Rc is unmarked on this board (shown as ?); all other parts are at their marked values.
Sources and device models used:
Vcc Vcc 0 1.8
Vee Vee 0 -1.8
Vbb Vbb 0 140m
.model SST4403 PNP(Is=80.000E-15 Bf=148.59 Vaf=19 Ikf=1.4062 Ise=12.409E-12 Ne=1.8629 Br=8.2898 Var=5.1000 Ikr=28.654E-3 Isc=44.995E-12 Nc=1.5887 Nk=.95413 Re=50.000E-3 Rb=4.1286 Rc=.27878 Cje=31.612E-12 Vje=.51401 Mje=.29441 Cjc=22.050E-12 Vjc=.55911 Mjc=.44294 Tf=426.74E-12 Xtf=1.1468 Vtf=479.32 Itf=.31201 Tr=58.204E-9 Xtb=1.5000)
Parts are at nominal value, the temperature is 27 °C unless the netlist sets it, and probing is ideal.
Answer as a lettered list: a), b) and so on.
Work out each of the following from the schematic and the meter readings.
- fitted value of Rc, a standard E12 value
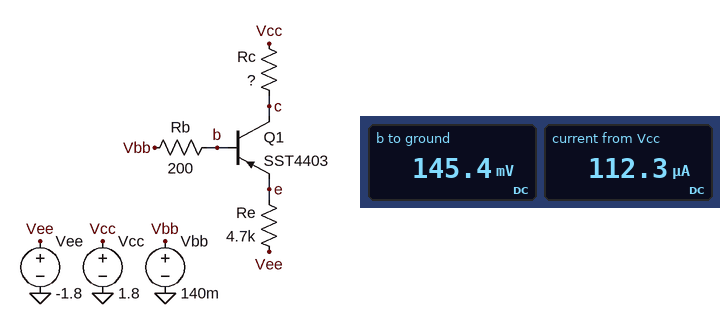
a) 10 kΩ
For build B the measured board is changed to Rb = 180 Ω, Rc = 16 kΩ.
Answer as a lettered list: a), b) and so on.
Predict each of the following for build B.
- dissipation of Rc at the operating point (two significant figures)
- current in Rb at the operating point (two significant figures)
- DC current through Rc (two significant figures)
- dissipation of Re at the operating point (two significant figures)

a) 81 µW
b) 18 µA
c) 71 µA
d) 13 µW
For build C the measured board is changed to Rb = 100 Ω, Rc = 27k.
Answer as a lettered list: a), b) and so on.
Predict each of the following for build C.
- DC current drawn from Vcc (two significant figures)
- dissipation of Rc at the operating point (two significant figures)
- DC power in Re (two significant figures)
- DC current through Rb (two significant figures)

a) 43 µA
b) 49 µW
c) 4.4 µW
d) 12 µA
